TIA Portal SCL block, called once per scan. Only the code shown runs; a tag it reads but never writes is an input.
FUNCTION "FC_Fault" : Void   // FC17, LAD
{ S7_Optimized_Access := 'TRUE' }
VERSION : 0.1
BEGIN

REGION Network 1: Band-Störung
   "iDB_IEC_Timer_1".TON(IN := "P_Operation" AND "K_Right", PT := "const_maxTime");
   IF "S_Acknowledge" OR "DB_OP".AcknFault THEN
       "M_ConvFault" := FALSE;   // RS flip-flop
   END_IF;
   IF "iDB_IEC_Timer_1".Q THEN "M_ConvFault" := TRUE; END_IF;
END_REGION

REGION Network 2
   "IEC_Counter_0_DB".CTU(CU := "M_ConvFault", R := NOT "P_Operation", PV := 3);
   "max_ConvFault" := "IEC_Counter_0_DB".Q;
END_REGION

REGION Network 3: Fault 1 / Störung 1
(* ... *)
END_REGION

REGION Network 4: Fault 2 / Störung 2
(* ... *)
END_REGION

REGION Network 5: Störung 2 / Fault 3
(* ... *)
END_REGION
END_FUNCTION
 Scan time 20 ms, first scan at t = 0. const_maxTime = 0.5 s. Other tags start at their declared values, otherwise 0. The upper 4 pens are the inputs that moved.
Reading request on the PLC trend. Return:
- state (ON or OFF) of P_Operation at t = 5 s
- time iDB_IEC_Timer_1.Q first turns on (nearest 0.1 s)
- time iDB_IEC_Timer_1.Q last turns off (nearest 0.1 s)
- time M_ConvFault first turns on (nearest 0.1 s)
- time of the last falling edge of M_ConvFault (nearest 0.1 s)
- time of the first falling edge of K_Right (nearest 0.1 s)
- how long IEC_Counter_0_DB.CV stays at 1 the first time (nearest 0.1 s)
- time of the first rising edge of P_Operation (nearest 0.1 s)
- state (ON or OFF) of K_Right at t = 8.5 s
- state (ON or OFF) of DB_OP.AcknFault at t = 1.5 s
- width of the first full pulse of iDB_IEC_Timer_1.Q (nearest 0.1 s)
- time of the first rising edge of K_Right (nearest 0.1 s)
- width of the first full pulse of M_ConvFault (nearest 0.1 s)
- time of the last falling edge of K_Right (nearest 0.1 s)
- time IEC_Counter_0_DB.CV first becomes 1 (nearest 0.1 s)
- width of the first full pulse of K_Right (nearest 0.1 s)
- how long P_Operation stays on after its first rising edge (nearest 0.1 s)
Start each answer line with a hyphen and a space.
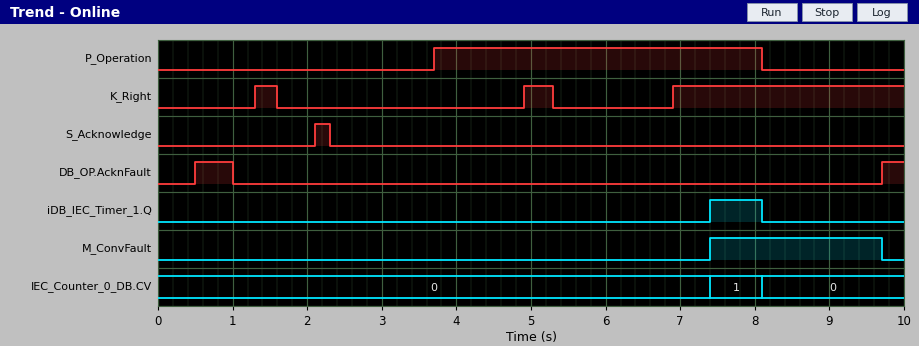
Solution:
- ON
- 7.4 s
- 8.1 s
- 7.4 s
- 9.7 s
- 1.6 s
- 0.7 s
- 3.7 s
- ON
- OFF
- 0.7 s
- 1.3 s
- 2.3 s
- 5.3 s
- 7.4 s
- 0.3 s
- 4.4 s
